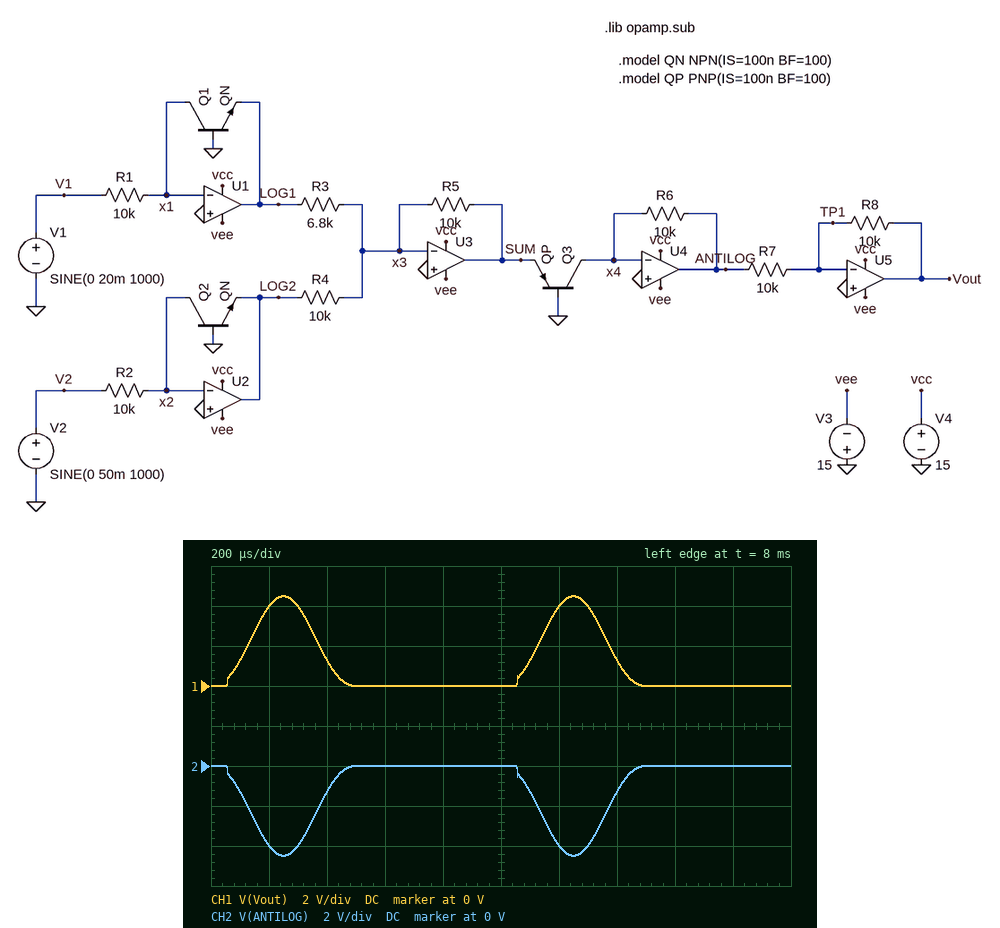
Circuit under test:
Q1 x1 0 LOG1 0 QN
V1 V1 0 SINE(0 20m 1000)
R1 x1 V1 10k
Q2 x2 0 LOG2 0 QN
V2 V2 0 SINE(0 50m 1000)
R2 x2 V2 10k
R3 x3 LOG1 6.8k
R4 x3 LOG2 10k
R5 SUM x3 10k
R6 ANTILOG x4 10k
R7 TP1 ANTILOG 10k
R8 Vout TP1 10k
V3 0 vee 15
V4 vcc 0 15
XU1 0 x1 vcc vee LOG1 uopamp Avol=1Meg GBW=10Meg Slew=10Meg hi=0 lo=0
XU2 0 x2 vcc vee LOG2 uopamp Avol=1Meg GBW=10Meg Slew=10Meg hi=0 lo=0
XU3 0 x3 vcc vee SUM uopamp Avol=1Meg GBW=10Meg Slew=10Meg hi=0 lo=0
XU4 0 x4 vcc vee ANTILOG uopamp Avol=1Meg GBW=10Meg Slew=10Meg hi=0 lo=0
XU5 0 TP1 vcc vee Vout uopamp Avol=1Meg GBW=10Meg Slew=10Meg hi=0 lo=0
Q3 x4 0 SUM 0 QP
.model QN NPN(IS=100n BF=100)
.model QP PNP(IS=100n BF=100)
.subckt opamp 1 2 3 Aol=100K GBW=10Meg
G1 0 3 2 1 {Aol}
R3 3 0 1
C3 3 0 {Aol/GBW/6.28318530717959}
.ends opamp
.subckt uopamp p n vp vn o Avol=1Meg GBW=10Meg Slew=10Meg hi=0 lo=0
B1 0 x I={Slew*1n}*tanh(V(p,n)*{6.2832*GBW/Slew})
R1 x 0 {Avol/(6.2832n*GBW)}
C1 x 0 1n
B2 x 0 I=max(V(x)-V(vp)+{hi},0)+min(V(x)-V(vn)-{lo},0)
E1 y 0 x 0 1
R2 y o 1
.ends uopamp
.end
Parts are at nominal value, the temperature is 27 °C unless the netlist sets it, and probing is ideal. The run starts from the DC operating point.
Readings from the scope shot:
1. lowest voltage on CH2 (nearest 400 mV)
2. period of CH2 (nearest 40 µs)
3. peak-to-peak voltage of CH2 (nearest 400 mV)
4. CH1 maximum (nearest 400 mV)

-4.4 V
1.00 ms
4.4 V
4.4 V
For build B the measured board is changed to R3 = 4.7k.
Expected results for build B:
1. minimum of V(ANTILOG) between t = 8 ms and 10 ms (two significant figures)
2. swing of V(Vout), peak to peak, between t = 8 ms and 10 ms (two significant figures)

-15 V
15 V
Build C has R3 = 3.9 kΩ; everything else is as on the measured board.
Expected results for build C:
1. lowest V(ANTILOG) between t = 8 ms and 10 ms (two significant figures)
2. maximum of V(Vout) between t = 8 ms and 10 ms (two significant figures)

-15 V
15 V
